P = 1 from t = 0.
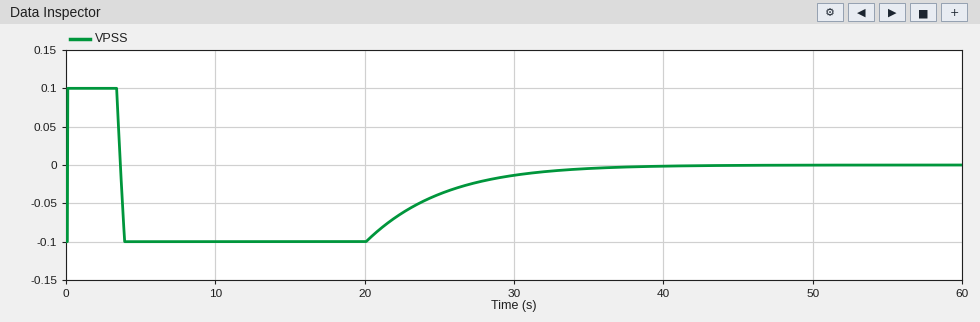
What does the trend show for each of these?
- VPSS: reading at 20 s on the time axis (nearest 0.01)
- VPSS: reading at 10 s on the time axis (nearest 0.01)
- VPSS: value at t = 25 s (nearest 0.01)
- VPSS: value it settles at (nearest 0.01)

-0.10
-0.10
-0.04
0.00
